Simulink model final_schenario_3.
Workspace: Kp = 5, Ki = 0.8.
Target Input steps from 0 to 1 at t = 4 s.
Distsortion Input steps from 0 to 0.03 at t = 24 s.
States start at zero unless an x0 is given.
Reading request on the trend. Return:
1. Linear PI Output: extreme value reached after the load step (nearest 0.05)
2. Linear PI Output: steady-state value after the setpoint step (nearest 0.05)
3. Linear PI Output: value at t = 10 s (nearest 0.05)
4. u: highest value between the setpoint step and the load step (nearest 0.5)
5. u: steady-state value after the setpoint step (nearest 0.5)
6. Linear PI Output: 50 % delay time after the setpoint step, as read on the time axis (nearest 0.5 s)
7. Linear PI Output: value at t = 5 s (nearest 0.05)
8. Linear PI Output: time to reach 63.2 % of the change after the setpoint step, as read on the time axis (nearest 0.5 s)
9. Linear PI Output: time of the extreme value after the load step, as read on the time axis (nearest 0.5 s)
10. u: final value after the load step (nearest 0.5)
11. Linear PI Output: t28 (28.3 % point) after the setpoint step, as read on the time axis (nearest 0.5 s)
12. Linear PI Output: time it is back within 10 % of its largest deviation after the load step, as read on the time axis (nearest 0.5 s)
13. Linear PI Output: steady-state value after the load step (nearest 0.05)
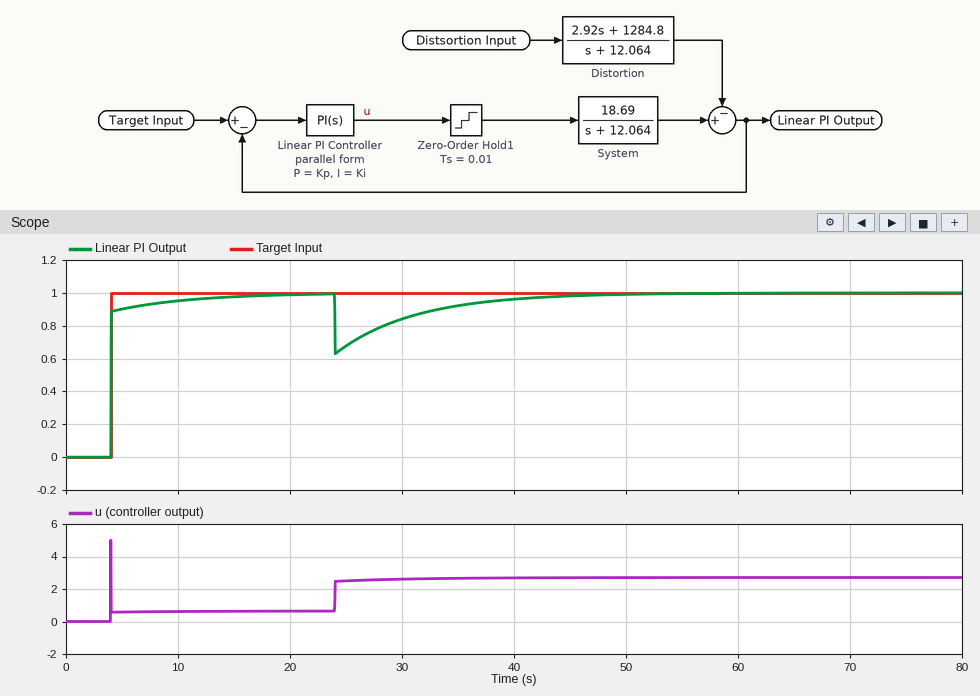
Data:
0.65
1.00
0.95
5.0
0.5
4.0 s
0.90
4.0 s
24.0 s
2.5
4.0 s
40.5 s
1.00
